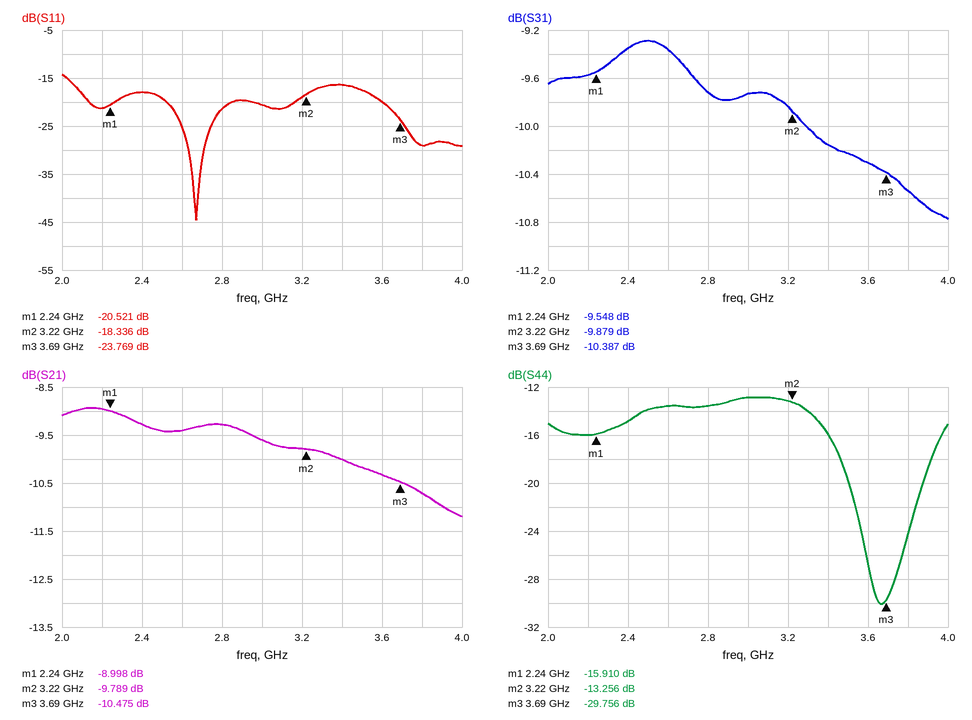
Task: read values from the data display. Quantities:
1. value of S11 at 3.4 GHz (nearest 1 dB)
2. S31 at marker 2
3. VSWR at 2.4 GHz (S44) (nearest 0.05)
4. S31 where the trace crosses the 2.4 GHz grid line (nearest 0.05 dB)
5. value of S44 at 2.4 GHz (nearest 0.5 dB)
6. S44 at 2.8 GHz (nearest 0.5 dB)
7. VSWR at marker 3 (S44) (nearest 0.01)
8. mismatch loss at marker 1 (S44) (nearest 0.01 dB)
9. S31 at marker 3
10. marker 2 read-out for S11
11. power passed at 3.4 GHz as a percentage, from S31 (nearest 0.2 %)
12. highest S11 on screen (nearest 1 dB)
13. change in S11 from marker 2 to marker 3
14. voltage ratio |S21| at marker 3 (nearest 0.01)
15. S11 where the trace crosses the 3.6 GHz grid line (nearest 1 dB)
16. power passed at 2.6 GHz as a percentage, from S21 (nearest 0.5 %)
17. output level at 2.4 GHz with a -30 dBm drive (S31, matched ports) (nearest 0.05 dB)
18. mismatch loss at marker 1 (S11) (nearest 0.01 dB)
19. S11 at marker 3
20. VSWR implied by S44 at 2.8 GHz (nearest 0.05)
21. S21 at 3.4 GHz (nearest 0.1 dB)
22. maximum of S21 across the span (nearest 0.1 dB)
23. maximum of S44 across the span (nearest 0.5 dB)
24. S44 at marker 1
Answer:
-16 dB
-9.879 dB
1.45
-9.35 dB
-15.0 dB
-13.5 dB
1.07
0.11 dB
-10.387 dB
-18.336 dB
9.6 %
-14 dB
-5.433 dB
0.30
-20 dB
11.5 %
-39.35 dBm
0.04 dB
-23.769 dB
1.55
-10.0 dB
-8.9 dB
-13.0 dB
-15.910 dB
